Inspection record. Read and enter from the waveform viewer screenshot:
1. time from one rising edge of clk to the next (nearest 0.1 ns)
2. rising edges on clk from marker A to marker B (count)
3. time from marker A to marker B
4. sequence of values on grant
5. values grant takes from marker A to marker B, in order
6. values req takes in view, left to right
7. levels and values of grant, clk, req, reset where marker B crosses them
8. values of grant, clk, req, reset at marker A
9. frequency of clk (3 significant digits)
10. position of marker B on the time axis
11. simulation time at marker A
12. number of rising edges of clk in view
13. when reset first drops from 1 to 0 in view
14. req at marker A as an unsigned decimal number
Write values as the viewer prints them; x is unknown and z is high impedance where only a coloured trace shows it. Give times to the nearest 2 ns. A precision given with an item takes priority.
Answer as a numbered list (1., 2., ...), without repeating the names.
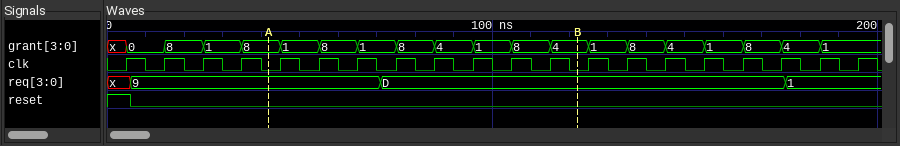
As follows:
1. 10 ns
2. 8
3. 80 ns
4. x, 0, 8, 1, 8, 1, 8, 1, 8, 4, 1, 8, 4, 1, 8, 4, 1, 8, 4, 1
5. 8, 1, 8, 1, 8, 4, 1, 8, 4
6. x, 9, D, 1
7. grant=4, clk=0, req=D, reset=0
8. grant=8, clk=0, req=9, reset=0
9. 100 MHz
10. 122 ns
11. 42 ns
12. 20
13. 6 ns
14. 9
